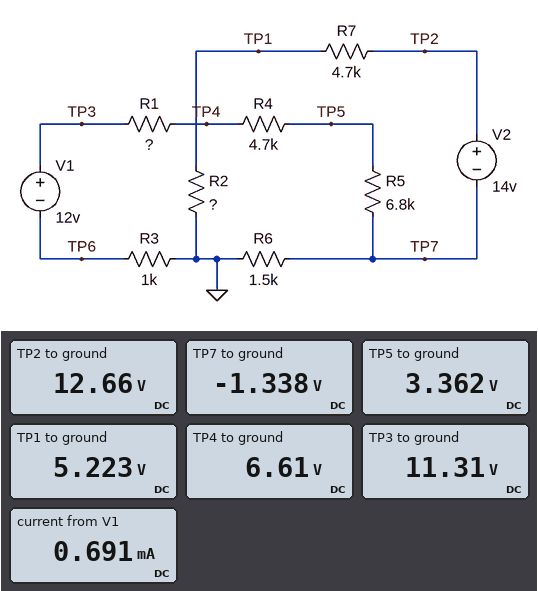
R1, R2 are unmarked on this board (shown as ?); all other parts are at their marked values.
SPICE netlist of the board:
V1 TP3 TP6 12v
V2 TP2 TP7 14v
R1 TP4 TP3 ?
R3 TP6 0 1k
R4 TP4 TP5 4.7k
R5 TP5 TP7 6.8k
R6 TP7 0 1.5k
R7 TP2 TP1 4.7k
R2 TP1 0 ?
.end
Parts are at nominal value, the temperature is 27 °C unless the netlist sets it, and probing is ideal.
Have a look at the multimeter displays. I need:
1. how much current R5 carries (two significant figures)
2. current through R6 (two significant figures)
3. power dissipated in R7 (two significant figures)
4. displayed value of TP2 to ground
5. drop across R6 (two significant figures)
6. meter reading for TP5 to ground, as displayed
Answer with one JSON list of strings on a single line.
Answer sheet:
["690 µA", "890 µA", "12 mW", "12.66 V", "1.3 V", "3.362 V"]
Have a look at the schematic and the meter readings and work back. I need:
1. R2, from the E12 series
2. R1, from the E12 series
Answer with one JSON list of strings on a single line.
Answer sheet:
["3.3 kΩ", "6.8 kΩ"]
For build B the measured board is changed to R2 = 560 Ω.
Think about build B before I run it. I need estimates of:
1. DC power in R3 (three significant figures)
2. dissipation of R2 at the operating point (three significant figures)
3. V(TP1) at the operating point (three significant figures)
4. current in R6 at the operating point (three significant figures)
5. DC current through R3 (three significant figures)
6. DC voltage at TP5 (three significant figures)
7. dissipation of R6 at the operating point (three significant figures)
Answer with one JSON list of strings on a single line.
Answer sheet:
["545 µW", "2.80 mW", "1.25 V", "1.50 mA", "738 µA", "2.77 V", "3.36 mW"]
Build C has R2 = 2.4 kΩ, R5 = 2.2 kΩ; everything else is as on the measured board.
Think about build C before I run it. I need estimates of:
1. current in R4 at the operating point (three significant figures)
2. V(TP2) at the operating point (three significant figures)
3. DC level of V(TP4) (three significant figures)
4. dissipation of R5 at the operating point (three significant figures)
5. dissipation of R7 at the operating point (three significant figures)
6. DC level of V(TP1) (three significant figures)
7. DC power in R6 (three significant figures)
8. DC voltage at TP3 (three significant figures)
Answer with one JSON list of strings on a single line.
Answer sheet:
["906 µA", "12.7 V", "4.93 V", "1.81 mW", "15.0 mW", "4.29 V", "1.16 mW", "11.1 V"]
